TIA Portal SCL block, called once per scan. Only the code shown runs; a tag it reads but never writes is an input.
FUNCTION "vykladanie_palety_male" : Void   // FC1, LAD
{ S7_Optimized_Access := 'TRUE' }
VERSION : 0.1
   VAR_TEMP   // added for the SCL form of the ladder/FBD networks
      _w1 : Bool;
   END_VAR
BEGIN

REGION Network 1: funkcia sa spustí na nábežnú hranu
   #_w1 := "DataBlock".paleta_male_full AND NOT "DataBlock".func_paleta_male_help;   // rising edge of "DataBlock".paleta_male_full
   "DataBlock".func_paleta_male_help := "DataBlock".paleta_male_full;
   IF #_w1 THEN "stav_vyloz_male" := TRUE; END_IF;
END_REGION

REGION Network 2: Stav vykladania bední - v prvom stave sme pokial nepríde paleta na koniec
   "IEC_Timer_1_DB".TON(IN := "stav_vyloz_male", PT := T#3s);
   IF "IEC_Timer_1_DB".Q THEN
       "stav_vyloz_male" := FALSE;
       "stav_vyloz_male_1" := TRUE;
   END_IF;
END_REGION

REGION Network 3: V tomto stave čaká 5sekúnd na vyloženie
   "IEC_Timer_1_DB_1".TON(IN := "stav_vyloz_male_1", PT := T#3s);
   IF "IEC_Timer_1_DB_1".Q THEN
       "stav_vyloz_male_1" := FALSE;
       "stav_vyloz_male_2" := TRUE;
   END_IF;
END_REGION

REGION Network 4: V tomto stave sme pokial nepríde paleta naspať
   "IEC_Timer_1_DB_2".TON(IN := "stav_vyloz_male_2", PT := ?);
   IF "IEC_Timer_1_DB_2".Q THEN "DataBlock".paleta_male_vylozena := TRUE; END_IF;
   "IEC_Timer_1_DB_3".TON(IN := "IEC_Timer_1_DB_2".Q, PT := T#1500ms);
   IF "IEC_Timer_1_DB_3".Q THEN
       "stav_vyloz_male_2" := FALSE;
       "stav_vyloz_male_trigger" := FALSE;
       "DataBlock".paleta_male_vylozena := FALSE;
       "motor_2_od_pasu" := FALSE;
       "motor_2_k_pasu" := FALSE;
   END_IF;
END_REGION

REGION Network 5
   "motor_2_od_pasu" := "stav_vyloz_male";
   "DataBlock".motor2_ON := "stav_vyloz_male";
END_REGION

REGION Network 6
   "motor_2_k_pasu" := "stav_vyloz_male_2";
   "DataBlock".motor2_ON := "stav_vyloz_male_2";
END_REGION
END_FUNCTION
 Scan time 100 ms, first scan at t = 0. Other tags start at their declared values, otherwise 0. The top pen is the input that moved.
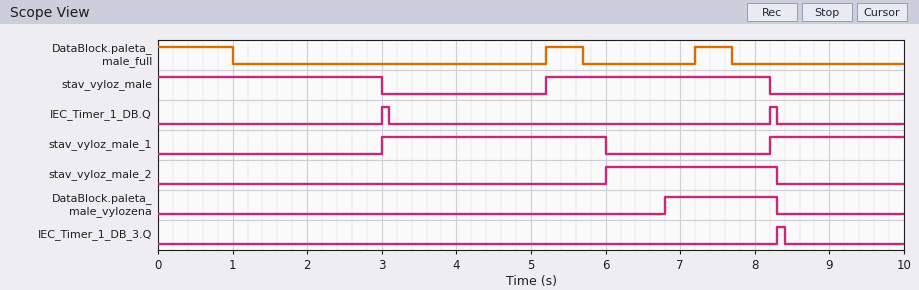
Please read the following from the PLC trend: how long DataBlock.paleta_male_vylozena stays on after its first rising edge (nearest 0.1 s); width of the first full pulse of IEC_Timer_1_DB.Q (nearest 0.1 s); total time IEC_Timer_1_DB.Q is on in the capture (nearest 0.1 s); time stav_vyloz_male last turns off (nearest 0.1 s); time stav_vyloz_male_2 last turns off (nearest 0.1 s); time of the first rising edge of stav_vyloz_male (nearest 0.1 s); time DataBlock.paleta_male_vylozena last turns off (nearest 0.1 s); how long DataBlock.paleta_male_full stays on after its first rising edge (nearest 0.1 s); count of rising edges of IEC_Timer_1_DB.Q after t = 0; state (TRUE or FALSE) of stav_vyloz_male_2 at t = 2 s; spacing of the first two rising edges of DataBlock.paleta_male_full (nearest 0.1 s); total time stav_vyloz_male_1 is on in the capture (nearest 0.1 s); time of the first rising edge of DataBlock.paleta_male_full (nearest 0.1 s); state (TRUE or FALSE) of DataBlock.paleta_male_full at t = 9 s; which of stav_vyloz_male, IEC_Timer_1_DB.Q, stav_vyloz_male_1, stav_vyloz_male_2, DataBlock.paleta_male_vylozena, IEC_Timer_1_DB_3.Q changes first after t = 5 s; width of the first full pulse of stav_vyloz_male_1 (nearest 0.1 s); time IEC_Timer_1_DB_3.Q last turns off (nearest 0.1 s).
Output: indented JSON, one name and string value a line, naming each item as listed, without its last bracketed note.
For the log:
{
  "how long DataBlock.paleta_male_vylozena stays on after its first rising edge": "1.5 s",
  "width of the first full pulse of IEC_Timer_1_DB.Q": "0.1 s",
  "total time IEC_Timer_1_DB.Q is on in the capture": "0.2 s",
  "time stav_vyloz_male last turns off": "8.2 s",
  "time stav_vyloz_male_2 last turns off": "8.3 s",
  "time of the first rising edge of stav_vyloz_male": "5.2 s",
  "time DataBlock.paleta_male_vylozena last turns off": "8.3 s",
  "how long DataBlock.paleta_male_full stays on after its first rising edge": "0.5 s",
  "count of rising edges of IEC_Timer_1_DB.Q after t = 0": "2",
  "state (TRUE or FALSE) of stav_vyloz_male_2 at t = 2 s": "FALSE",
  "spacing of the first two rising edges of DataBlock.paleta_male_full": "2.0 s",
  "total time stav_vyloz_male_1 is on in the capture": "4.8 s",
  "time of the first rising edge of DataBlock.paleta_male_full": "5.2 s",
  "state (TRUE or FALSE) of DataBlock.paleta_male_full at t = 9 s": "FALSE",
  "which of stav_vyloz_male, IEC_Timer_1_DB.Q, stav_vyloz_male_1, stav_vyloz_male_2, DataBlock.paleta_male_vylozena, IEC_Timer_1_DB_3.Q changes first after t = 5 s": "stav_vyloz_male",
  "width of the first full pulse of stav_vyloz_male_1": "3.0 s",
  "time IEC_Timer_1_DB_3.Q last turns off": "8.4 s"
}
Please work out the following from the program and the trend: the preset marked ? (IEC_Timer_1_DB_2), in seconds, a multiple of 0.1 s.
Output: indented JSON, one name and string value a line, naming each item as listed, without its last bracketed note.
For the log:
{
  "the preset marked ? (IEC_Timer_1_DB_2), in seconds, a multiple of 0.1 s": "0.8 s"
}
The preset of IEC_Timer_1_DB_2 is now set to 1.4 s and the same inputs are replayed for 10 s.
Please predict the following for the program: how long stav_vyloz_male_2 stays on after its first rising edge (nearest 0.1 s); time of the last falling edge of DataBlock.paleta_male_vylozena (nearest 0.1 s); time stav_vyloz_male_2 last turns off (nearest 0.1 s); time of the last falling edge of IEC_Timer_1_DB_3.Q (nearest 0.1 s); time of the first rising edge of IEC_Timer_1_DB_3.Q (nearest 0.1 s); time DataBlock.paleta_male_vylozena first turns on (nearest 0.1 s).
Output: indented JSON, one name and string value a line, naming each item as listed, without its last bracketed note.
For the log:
{
  "how long stav_vyloz_male_2 stays on after its first rising edge": "2.9 s",
  "time of the last falling edge of DataBlock.paleta_male_vylozena": "8.9 s",
  "time stav_vyloz_male_2 last turns off": "8.9 s",
  "time of the last falling edge of IEC_Timer_1_DB_3.Q": "9.0 s",
  "time of the first rising edge of IEC_Timer_1_DB_3.Q": "8.9 s",
  "time DataBlock.paleta_male_vylozena first turns on": "7.4 s"
}
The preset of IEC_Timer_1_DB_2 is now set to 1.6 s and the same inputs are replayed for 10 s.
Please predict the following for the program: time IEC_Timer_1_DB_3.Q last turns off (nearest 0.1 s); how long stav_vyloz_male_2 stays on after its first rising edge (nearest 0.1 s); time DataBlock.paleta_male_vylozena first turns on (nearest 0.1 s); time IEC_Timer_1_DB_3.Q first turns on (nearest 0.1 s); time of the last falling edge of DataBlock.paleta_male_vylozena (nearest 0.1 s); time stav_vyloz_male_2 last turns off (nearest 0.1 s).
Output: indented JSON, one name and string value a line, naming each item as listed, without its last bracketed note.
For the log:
{
  "time IEC_Timer_1_DB_3.Q last turns off": "9.2 s",
  "how long stav_vyloz_male_2 stays on after its first rising edge": "3.1 s",
  "time DataBlock.paleta_male_vylozena first turns on": "7.6 s",
  "time IEC_Timer_1_DB_3.Q first turns on": "9.1 s",
  "time of the last falling edge of DataBlock.paleta_male_vylozena": "9.1 s",
  "time stav_vyloz_male_2 last turns off": "9.1 s"
}
